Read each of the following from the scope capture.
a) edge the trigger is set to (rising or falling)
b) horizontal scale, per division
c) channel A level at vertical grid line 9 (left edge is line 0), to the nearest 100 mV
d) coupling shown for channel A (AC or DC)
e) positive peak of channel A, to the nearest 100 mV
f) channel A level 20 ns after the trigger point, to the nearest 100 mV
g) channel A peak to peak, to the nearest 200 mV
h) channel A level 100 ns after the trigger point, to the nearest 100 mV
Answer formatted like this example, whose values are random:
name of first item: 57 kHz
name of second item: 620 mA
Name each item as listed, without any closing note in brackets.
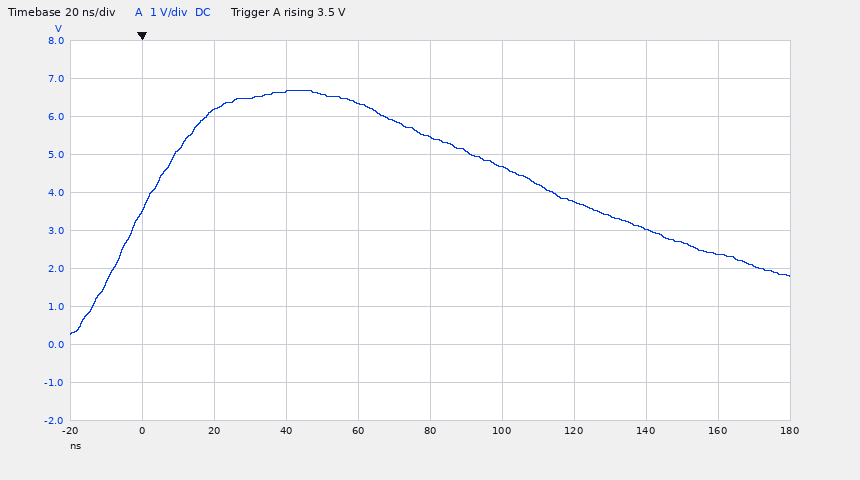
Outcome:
edge the trigger is set to: rising
horizontal scale, per division: 20 ns
channel A level at vertical grid line 9 (left edge is line 0), to the nearest 100 mV: 2.4 V
coupling shown for channel A: DC
positive peak of channel A, to the nearest 100 mV: 6.7 V
channel A level 20 ns after the trigger point, to the nearest 100 mV: 6.2 V
channel A peak to peak, to the nearest 200 mV: 6.4 V
channel A level 100 ns after the trigger point, to the nearest 100 mV: 4.7 V
